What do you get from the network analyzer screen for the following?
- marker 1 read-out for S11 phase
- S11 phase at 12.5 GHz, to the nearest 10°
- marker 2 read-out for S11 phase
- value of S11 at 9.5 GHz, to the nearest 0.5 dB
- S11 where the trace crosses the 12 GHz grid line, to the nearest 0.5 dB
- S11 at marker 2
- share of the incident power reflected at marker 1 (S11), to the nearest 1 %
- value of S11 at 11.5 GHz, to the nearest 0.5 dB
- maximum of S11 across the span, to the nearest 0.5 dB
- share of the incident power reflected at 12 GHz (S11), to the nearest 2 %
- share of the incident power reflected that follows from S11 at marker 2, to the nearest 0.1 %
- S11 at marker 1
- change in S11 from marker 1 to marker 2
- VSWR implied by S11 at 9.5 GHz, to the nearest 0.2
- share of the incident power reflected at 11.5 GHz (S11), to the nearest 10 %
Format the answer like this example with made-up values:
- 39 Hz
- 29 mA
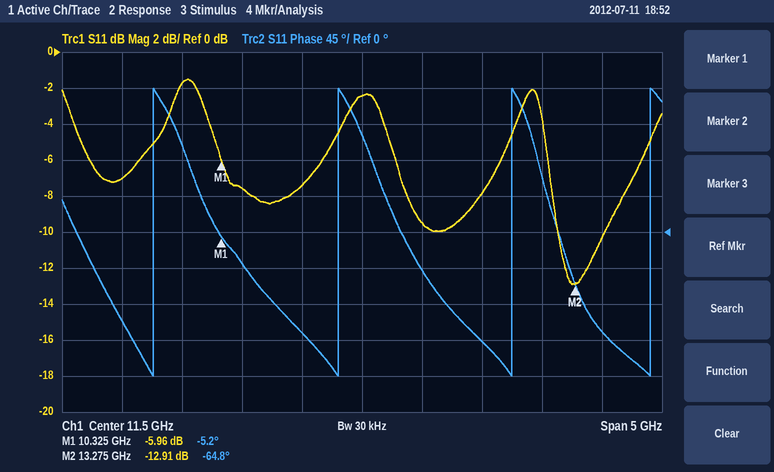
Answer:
- -5.2°
- -140°
- -64.8°
- -7.0 dB
- -9.5 dB
- -12.91 dB
- 25 %
- -2.5 dB
- -1.5 dB
- 12 %
- 5.1 %
- -5.96 dB
- -6.95 dB
- 2.6
- 60 %
